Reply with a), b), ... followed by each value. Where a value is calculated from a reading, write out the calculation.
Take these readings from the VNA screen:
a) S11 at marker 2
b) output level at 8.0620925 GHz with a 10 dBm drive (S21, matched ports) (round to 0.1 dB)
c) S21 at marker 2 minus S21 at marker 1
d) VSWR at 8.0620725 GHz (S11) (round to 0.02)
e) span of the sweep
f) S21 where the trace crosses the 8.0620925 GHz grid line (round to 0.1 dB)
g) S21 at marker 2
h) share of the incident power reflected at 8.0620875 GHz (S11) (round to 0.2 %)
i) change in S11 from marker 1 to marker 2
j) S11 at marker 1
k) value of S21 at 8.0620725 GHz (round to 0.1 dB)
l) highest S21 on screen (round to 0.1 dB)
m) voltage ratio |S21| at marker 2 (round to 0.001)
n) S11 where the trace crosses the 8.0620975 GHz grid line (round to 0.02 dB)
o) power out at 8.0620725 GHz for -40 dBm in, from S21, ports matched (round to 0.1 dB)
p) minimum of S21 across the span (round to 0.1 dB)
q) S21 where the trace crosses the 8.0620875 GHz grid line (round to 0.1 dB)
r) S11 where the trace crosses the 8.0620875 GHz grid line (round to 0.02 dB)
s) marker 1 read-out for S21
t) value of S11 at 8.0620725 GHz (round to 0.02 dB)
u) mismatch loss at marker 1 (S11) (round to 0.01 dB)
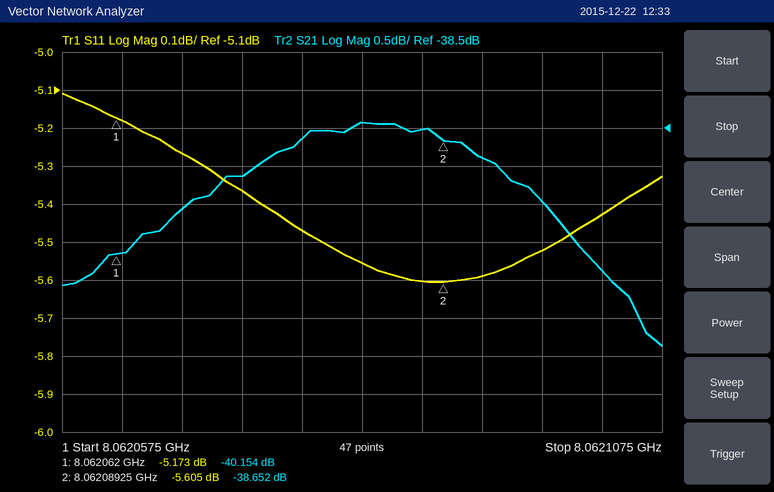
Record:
a) -5.605 dB
b) 10 dBm + (-38.9 dB) = -28.9 dBm
c) -38.652 − (-40.154) = 1.502 dB
d) |Γ| = 10^(-5.36/20) = 0.5395; VSWR = (1 + 0.5395)/(1 − 0.5395) ≈ 3.34
e) 50 kHz
f) -38.9 dB
g) -38.652 dB
h) 10^(-5.6/10) ≈ 27.5 %, so 27.6 % to the nearest 0.2 %
i) -5.605 − (-5.173) = -0.432 dB
j) -5.173 dB
k) -39.1 dB
l) -38.4 dB
m) 10^(-38.652/20) ≈ 0.012
n) -5.52 dB
o) -40 dBm + (-39.1 dB) = -79.1 dBm
p) -41.4 dB
q) -38.5 dB
r) -5.60 dB
s) -40.154 dB
t) -5.36 dB
u) −10 log10(1 − 10^(-5.173/10)) ≈ 1.57 dB
